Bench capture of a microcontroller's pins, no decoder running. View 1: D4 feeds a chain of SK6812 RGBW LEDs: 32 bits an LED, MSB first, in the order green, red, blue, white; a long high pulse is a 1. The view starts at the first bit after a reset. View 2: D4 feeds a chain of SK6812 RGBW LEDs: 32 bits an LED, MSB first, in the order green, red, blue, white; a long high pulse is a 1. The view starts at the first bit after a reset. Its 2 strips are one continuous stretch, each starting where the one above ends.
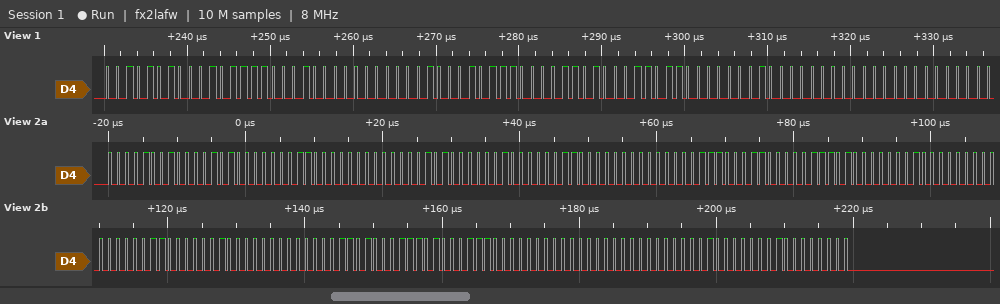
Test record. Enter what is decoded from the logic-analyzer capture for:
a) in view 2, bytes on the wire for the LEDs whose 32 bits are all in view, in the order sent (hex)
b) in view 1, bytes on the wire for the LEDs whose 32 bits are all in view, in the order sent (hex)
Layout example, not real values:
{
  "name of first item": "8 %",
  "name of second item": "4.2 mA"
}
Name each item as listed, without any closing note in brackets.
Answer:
{
  "in view 2, bytes on the wire for the LEDs whose 32 bits are all in view, in the order sent": "09 0A 03 00 05 02 06 00 07 18 3A 02 00 03 02 00 0D 1D 1C 00 00 01 01 00",
  "in view 1, bytes on the wire for the LEDs whose 32 bits are all in view, in the order sent": "2A 2F 10 01 17 0D 1B 01"
}
